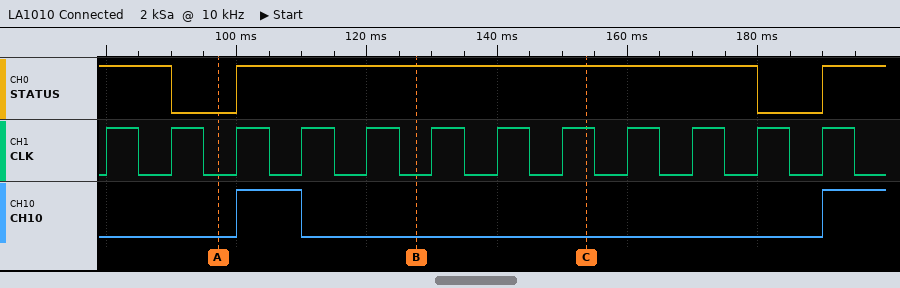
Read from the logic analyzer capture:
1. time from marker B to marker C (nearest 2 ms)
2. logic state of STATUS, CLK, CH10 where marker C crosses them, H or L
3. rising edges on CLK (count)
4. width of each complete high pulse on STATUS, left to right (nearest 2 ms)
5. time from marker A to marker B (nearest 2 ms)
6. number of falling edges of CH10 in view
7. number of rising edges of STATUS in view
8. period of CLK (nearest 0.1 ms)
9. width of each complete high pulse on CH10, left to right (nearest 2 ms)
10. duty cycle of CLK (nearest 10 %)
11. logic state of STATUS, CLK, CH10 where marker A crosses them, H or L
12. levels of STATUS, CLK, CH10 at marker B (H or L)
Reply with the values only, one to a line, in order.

26 ms
STATUS=H, CLK=H, CH10=L
12
80 ms
30 ms
1
2
10 ms
10 ms
50 %
STATUS=L, CLK=L, CH10=L
STATUS=H, CLK=L, CH10=L
